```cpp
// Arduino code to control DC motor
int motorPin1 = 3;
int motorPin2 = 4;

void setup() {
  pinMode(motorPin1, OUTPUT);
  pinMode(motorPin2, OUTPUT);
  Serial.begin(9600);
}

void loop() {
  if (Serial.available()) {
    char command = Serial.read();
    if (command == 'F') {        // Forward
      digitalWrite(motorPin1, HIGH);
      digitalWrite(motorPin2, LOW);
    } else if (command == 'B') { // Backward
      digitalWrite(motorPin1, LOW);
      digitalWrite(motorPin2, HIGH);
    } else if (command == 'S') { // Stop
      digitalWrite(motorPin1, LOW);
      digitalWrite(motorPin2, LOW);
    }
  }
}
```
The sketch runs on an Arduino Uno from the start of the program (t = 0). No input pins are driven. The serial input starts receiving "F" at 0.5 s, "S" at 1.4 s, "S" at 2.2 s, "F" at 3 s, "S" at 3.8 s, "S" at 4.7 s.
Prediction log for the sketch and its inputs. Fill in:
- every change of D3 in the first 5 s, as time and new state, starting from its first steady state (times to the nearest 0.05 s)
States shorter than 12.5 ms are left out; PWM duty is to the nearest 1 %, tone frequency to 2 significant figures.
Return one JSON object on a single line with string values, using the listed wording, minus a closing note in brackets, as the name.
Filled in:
{"every change of D3 in the first 5 s, as time and new state, starting from its first steady state": "0 s low; 0.5 s high; 1.4 s low; 3 s high; 3.8 s low"}
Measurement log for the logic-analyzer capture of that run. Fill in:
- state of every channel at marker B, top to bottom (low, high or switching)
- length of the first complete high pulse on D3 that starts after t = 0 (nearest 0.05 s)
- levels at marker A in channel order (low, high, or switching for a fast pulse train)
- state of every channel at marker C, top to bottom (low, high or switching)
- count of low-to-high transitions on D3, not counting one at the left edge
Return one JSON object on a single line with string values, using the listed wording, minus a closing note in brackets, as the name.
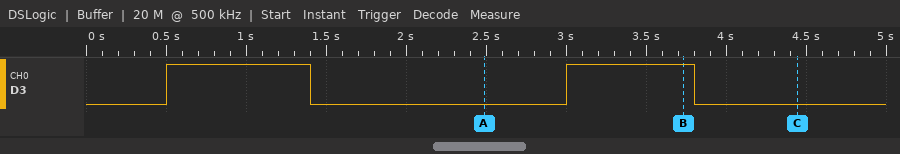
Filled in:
{"state of every channel at marker B, top to bottom": "D3 high", "length of the first complete high pulse on D3 that starts after t = 0": "0.90 s", "levels at marker A in channel order": "D3 low", "state of every channel at marker C, top to bottom": "D3 low", "count of low-to-high transitions on D3, not counting one at the left edge": "2"}
